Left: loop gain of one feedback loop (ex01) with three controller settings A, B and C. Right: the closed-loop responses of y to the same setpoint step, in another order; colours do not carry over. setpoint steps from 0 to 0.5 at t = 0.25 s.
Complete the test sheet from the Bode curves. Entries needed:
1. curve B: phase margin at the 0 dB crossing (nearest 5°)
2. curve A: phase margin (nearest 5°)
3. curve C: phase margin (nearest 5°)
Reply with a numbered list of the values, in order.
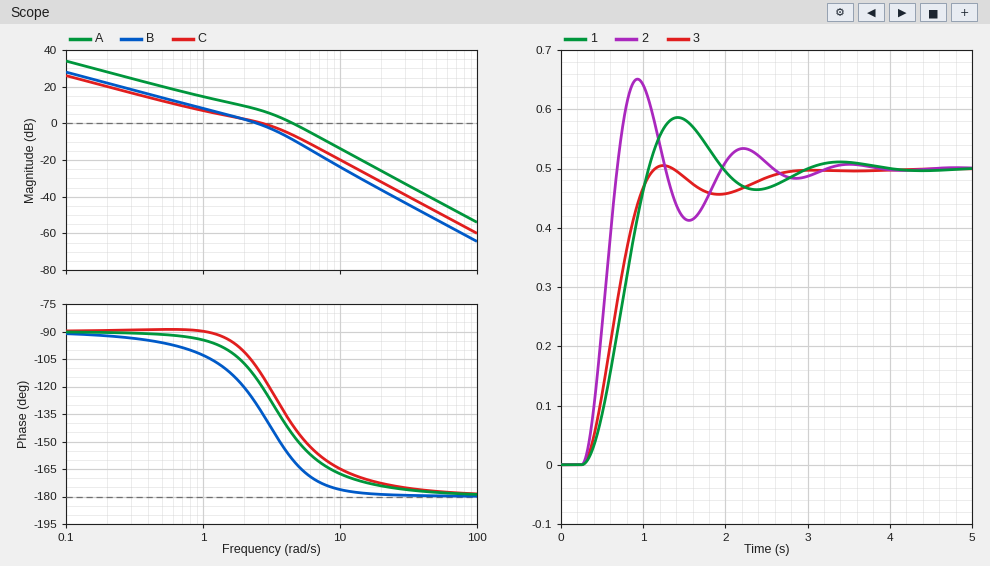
1. 50°
2. 35°
3. 65°
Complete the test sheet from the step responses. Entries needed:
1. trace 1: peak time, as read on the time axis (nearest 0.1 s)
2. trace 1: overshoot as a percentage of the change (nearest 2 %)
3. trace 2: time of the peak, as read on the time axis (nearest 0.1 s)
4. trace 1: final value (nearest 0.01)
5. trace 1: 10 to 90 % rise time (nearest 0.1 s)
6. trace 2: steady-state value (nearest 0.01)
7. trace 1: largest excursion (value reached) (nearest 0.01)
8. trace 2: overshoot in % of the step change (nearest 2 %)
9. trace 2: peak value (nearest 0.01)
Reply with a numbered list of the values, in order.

1. 1.4 s
2. 18 %
3. 0.9 s
4. 0.50
5. 0.5 s
6. 0.50
7. 0.59
8. 30 %
9. 0.65
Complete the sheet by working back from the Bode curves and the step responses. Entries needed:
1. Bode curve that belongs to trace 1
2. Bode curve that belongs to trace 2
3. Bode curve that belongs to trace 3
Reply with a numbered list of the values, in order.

1. B
2. A
3. C
